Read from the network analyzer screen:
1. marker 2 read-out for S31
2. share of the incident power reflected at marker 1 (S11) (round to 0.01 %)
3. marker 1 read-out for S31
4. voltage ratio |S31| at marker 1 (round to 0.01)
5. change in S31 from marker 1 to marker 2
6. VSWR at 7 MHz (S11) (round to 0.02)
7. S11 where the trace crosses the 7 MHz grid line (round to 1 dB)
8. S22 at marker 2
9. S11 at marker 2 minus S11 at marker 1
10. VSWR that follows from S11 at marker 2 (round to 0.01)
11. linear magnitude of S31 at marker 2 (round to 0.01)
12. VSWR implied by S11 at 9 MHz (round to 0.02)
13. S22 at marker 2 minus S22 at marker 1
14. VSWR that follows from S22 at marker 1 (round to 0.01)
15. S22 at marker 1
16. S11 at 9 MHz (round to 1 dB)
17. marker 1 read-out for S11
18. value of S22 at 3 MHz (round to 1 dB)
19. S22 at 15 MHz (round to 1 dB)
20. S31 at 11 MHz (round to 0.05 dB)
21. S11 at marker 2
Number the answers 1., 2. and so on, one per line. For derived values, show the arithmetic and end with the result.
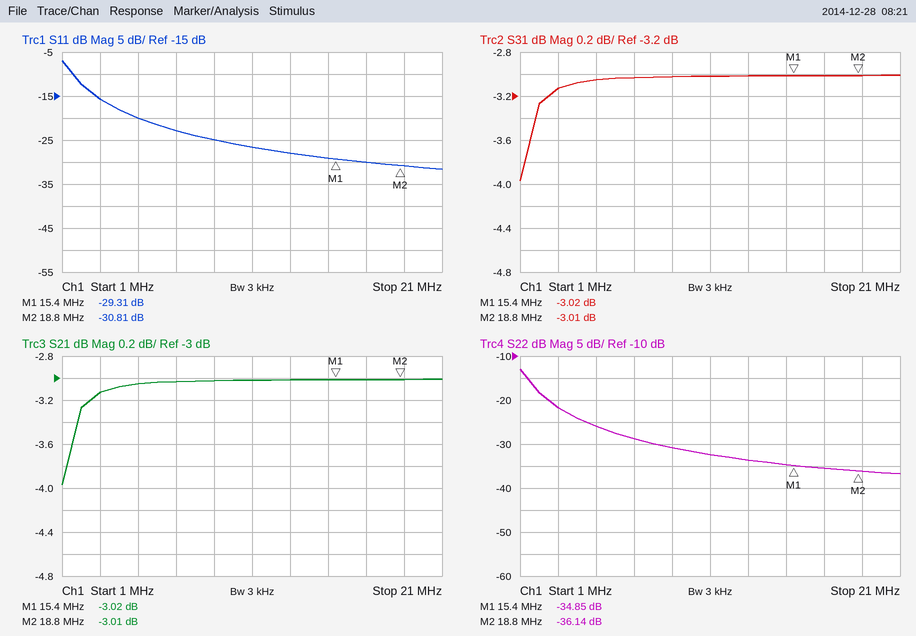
1. -3.01 dB
2. 10^(-29.31/10) ≈ 0.12 %
3. -3.02 dB
4. 10^(-3.02/20) ≈ 0.71
5. -3.01 − (-3.02) = 0.01 dB
6. |Γ| = 10^(-23/20) = 0.0708; VSWR = (1 + 0.0708)/(1 − 0.0708) ≈ 1.15, so 1.16 to the nearest 0.02
7. -23 dB
8. -36.14 dB
9. -30.81 − (-29.31) = -1.50 dB
10. (1 + 0.0288)/(1 − 0.0288) ≈ 1.06
11. 10^(-3.01/20) ≈ 0.71
12. |Γ| = 10^(-25/20) = 0.0562; VSWR = (1 + 0.0562)/(1 − 0.0562) ≈ 1.12
13. -36.14 − (-34.85) = -1.29 dB
14. (1 + 0.0181)/(1 − 0.0181) ≈ 1.04
15. -34.85 dB
16. -25 dB
17. -29.31 dB
18. -22 dB
19. -35 dB
20. -3.00 dB
21. -30.81 dB
